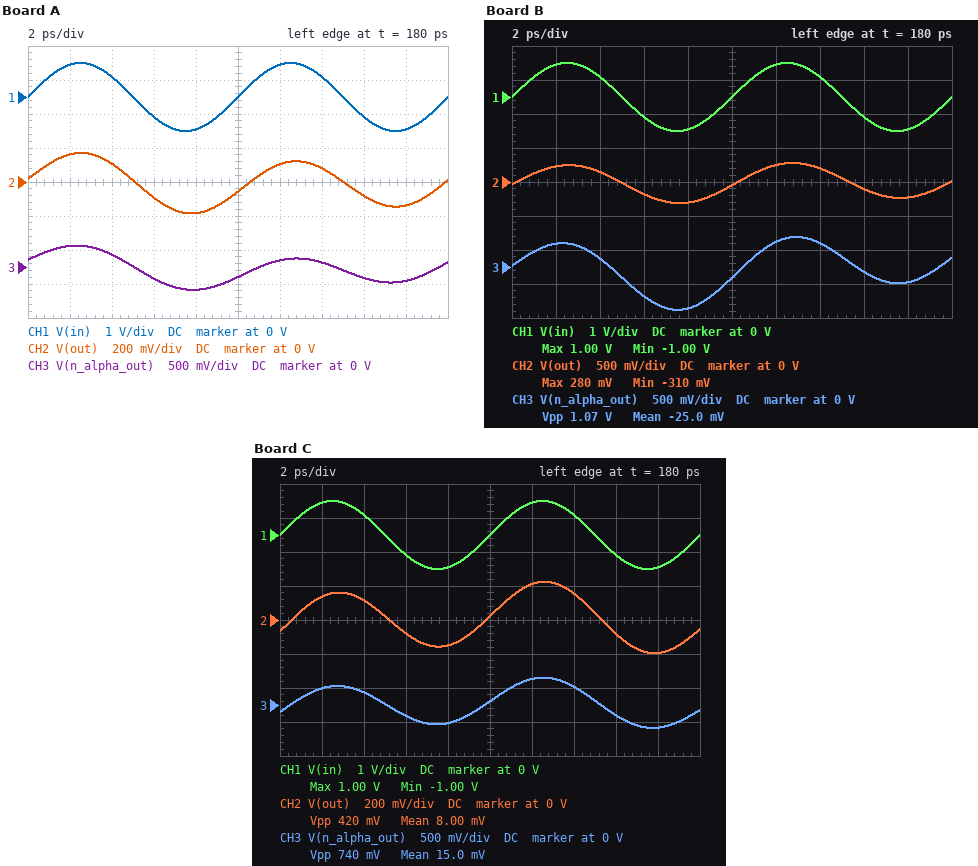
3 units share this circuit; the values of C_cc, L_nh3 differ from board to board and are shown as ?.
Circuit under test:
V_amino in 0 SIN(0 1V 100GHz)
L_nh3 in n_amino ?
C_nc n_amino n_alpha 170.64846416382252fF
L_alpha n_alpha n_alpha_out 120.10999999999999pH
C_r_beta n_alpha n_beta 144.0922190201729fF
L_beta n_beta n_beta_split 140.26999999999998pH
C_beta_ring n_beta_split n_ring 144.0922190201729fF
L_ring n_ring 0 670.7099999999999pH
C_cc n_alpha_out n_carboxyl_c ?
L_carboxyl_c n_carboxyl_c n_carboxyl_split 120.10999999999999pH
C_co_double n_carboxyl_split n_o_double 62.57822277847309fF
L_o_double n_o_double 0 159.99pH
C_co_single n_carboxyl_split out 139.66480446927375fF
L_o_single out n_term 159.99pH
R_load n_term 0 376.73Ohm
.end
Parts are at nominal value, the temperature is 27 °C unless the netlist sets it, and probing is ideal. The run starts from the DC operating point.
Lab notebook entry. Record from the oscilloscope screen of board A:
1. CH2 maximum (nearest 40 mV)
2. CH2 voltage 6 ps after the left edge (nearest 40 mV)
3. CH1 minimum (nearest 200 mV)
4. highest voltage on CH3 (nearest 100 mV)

160 mV
-80 mV
-1.0 V
300 mV
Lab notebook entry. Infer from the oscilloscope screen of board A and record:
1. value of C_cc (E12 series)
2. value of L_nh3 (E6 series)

47 fF
330 pH
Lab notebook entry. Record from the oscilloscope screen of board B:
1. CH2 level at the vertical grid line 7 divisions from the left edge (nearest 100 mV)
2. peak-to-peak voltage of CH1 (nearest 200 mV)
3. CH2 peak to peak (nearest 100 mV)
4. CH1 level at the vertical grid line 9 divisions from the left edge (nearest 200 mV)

200 mV
2.0 V
600 mV
-1.0 V
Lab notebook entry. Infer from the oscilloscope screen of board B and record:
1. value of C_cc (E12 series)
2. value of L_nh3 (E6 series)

47 fF
100 pH
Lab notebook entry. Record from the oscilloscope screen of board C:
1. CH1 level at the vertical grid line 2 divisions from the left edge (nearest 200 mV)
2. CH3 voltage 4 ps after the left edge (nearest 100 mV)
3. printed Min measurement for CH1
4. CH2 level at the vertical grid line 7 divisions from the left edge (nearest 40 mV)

600 mV
200 mV
-1.00 V
160 mV
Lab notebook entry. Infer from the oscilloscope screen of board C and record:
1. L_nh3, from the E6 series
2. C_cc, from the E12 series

220 pH
82 fF
